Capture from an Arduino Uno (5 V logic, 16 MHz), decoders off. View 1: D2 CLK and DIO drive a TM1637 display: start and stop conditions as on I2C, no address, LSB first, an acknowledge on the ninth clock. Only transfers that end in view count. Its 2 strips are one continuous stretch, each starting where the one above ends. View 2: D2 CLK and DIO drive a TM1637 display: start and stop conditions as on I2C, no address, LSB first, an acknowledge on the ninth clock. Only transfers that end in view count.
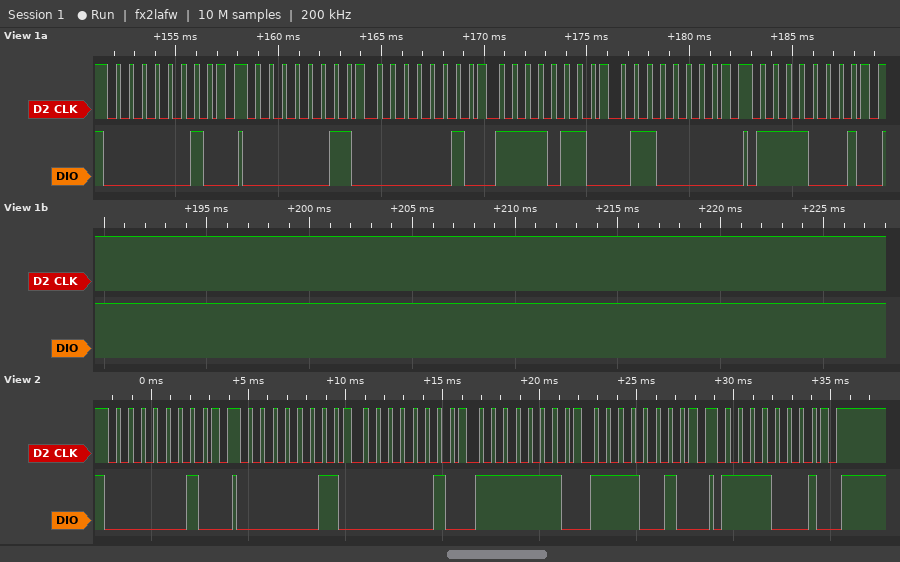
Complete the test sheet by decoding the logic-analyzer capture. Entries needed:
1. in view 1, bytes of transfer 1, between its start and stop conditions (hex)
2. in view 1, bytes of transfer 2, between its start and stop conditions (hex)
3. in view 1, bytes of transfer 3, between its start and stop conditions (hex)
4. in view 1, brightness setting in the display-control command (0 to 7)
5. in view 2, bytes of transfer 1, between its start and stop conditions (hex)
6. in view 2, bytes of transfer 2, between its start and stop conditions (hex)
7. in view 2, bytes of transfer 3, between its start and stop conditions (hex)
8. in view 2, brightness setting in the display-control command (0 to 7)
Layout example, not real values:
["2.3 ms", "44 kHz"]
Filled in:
["40", "C0 40 6F 06", "8F", "7", "40", "C0 40 7F 4F", "8F", "7"]
